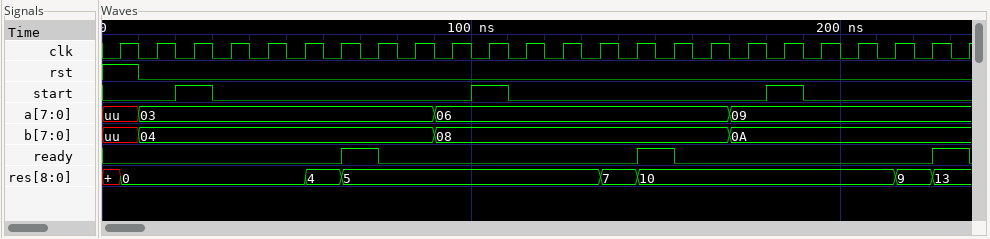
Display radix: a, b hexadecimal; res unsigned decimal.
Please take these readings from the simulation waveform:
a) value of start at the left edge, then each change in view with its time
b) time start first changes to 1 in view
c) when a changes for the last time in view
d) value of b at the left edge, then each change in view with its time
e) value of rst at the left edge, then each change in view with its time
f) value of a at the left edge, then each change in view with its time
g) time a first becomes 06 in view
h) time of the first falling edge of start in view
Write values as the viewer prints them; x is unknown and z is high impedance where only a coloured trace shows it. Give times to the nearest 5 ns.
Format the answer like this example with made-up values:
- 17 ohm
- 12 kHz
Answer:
- 0, 1 at 20 ns, 0 at 30 ns, 1 at 100 ns, 0 at 110 ns, 1 at 180 ns, 0 at 190 ns
- 20 ns
- 170 ns
- uu, 04 at 10 ns, 08 at 90 ns, 0A at 170 ns
- 1, 0 at 10 ns
- uu, 03 at 10 ns, 06 at 90 ns, 09 at 170 ns
- 90 ns
- 30 ns
